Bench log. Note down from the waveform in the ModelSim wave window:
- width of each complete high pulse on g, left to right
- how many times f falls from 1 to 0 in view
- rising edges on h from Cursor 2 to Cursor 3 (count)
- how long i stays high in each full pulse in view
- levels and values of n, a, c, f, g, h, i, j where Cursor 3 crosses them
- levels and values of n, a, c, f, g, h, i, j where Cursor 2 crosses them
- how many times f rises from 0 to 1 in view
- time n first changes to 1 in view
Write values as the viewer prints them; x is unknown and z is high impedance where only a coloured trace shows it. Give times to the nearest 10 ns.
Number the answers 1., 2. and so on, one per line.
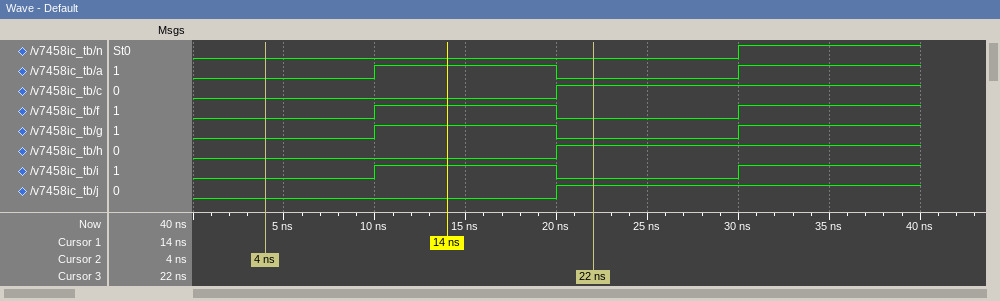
1. 10 ns
2. 1
3. 1
4. 10 ns
5. n=0, a=0, c=1, f=0, g=0, h=1, i=0, j=1
6. n=0, a=0, c=0, f=0, g=0, h=0, i=0, j=0
7. 2
8. 30 ns
